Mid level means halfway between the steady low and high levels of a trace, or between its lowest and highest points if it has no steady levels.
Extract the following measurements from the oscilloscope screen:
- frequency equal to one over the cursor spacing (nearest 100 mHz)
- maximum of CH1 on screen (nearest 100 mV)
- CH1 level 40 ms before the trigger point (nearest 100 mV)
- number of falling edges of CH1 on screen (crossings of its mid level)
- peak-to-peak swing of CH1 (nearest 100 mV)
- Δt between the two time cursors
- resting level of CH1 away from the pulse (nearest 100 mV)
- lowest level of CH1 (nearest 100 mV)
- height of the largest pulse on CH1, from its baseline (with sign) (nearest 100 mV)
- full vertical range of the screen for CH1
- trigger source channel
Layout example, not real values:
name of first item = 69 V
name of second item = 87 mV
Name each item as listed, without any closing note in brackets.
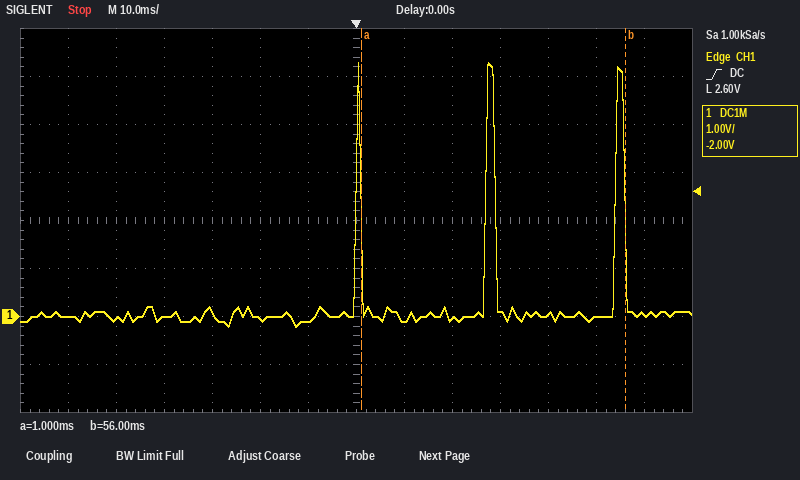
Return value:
frequency equal to one over the cursor spacing = 18.2 Hz
maximum of CH1 on screen = 5.3 V
CH1 level 40 ms before the trigger point = 0.0 V
number of falling edges of CH1 on screen = 3
peak-to-peak swing of CH1 = 5.5 V
Δt between the two time cursors = 55 ms
resting level of CH1 away from the pulse = 0.0 V
lowest level of CH1 = -200 mV
height of the largest pulse on CH1, from its baseline (with sign) = +5.3 V
full vertical range of the screen for CH1 = 8 V
trigger source channel = CH1
